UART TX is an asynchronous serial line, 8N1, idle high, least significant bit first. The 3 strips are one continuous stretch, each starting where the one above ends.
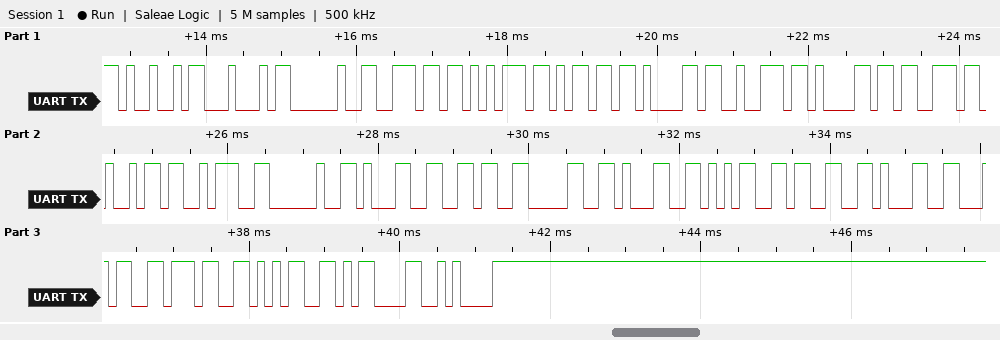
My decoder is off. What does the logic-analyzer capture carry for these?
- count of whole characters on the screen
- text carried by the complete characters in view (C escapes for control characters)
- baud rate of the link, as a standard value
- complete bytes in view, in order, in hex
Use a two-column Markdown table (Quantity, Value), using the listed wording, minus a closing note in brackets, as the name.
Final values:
| Quantity | Value |
|---|---|
| count of whole characters on the screen | 25 |
| text carried by the complete characters in view | "ID numarasi: 1601531475\r\n" |
| baud rate of the link, as a standard value | 9600 baud |
| complete bytes in view, in order, in hex | 0x49 0x44 0x20 0x6E 0x75 0x6D 0x61 0x72 0x61 0x73 0x69 0x3A 0x20 0x31 0x36 0x30 0x31 0x35 0x33 0x31 0x34 0x37 0x35 0x0D 0x0A |
